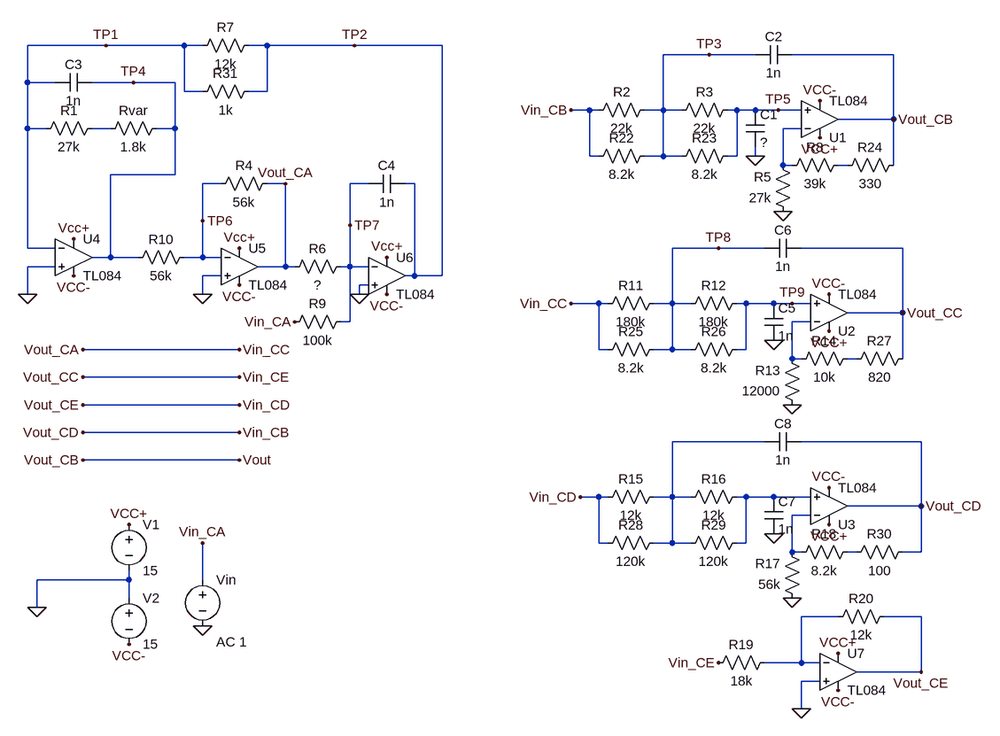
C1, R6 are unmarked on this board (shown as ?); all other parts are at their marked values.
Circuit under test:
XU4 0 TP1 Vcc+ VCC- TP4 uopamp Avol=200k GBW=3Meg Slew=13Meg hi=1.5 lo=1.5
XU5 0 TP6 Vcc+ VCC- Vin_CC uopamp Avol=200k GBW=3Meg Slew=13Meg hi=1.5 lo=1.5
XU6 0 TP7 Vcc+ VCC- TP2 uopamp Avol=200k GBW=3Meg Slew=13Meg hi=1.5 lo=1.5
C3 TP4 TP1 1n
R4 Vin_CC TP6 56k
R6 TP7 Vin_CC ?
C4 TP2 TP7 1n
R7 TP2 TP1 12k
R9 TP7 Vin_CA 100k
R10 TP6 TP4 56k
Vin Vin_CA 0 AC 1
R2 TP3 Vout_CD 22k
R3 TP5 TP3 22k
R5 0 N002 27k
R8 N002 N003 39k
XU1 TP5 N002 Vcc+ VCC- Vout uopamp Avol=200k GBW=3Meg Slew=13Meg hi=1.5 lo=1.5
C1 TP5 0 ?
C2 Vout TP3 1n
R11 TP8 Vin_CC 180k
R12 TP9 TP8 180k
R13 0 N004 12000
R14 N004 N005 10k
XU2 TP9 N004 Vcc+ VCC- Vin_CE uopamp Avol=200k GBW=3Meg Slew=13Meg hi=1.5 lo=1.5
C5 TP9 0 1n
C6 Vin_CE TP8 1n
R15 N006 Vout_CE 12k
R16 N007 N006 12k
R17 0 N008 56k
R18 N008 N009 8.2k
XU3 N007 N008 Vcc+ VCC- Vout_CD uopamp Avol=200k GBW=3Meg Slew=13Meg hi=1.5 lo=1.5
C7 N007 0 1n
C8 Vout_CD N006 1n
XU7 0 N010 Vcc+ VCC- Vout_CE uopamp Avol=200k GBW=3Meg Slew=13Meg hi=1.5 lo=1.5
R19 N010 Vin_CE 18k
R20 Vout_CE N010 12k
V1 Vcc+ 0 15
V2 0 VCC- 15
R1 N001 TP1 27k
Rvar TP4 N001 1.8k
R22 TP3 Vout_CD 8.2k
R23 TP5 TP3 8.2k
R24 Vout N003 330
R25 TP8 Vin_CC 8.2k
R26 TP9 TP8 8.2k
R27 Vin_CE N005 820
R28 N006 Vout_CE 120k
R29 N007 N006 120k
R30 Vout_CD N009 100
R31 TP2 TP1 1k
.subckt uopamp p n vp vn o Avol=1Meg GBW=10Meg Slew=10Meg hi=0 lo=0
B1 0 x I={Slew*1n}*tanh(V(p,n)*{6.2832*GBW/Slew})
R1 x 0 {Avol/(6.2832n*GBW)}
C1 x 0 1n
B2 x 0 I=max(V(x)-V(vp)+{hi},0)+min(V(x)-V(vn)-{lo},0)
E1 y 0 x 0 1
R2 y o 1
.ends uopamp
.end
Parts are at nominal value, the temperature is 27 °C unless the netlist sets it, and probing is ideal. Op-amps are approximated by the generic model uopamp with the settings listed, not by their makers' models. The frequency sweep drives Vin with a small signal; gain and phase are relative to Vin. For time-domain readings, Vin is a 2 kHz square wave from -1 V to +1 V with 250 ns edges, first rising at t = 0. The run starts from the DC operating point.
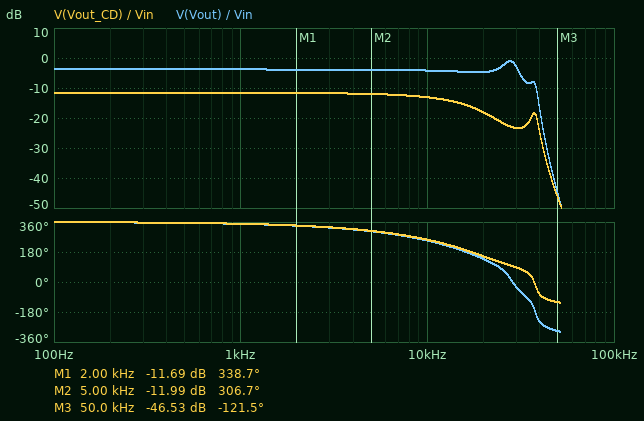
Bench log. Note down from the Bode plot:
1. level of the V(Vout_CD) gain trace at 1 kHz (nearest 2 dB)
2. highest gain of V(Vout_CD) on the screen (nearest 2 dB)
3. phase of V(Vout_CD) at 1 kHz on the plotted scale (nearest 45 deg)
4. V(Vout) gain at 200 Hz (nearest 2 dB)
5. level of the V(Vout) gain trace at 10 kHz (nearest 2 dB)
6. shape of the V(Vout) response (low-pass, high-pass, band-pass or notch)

-12 dB
-12 dB
360 deg
-4 dB
-4 dB
low-pass
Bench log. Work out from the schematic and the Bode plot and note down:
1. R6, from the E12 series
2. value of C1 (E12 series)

18 kΩ
820 pF
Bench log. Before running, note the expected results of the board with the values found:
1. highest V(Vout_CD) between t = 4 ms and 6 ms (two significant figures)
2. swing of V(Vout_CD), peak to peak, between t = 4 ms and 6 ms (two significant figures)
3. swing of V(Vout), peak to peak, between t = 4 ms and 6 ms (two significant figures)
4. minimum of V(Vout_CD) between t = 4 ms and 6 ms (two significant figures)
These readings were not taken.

280 mV
560 mV
1.7 V
-280 mV
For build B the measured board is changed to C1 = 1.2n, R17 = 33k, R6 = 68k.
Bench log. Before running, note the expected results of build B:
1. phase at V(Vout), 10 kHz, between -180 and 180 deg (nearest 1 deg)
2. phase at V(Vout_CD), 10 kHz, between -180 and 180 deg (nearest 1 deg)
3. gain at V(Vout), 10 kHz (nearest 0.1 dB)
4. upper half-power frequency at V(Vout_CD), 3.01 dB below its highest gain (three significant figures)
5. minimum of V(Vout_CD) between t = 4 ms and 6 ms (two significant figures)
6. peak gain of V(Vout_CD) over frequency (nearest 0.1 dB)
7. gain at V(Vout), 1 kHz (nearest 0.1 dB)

-137 deg
-113 deg
10.3 dB
20.6 kHz
-1.7 V
5.3 dB
8.5 dB
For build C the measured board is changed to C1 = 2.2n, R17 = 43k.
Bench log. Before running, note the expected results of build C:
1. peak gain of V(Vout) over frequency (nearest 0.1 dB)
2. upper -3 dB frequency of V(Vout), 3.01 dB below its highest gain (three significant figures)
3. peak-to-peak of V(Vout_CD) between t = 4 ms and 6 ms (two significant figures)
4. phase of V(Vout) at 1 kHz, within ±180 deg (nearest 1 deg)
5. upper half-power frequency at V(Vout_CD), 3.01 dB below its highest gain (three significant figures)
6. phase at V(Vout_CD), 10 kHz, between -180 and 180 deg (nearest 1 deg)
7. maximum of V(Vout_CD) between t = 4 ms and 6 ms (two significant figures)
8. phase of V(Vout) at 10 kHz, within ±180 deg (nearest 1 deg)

-3.5 dB
9.18 kHz
590 mV
-17 deg
14.6 kHz
-106 deg
290 mV
-165 deg
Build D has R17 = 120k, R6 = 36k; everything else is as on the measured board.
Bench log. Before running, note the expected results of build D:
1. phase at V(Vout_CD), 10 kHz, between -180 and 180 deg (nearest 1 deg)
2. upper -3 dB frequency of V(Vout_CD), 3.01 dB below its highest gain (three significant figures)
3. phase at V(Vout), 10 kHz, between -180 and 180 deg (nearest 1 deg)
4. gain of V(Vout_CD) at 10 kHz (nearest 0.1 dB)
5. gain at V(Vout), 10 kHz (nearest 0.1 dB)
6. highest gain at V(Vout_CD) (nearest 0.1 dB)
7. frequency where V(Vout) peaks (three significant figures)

-110 deg
27.7 kHz
-115 deg
-7.4 dB
1.6 dB
-6.2 dB
26.7 kHz
